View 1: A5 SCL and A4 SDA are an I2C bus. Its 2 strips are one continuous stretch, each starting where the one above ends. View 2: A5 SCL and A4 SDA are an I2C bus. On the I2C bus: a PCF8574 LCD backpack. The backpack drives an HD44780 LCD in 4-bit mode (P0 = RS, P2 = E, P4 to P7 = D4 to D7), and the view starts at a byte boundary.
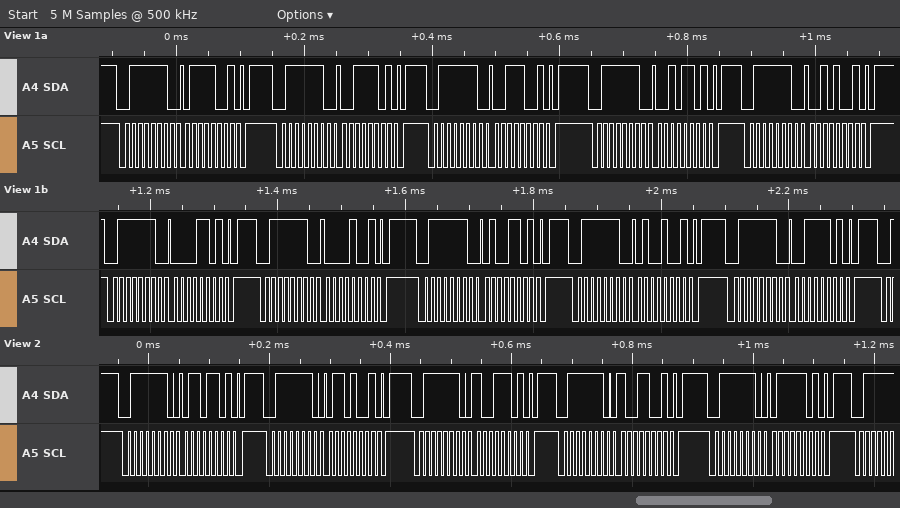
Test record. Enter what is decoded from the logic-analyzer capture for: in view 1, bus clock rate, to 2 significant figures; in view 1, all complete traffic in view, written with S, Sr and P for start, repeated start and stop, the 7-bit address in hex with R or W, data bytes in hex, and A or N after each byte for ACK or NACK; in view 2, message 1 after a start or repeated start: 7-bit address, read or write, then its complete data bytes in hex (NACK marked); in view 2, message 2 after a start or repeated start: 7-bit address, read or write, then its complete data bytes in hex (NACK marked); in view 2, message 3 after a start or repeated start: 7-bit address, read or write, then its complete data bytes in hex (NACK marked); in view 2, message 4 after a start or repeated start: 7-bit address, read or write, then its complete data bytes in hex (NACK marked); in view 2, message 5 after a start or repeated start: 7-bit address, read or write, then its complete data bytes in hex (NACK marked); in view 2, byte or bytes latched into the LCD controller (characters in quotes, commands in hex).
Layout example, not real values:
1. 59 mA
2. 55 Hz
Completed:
1. 100 kHz
2. S 3FW A 79 A P S 3FW A 3D A P S 3FW A 39 A P S 3FW A 2D A P S 3FW A 29 A P S 3FW A 0D A P S 3FW A 09 A P S 3FW A 4D A P S 3FW A 49 A P S 3FW A 3D A P
3. 0x3F write: 6D
4. 0x3F write: 69
5. 0x3F write: 9D
6. 0x3F write: 99
7. 0x3F write: 7D
8. 'i'
